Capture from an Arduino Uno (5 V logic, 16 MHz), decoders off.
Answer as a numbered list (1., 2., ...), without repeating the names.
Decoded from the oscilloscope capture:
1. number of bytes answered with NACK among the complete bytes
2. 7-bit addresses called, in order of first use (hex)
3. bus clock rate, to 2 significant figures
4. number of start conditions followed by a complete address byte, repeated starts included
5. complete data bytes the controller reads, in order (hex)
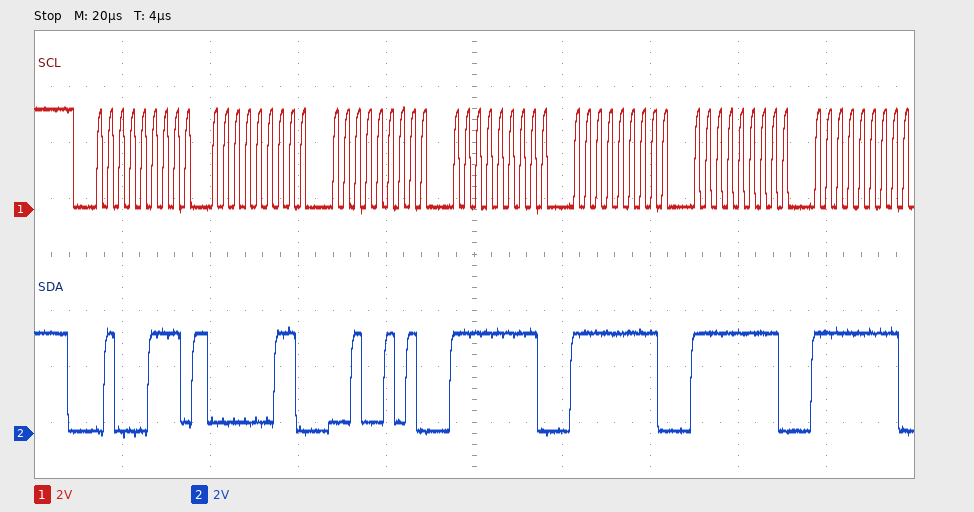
1. 0
2. 0x23
3. 400 kHz
4. 1
5. 03 25 FF FF FF FF
